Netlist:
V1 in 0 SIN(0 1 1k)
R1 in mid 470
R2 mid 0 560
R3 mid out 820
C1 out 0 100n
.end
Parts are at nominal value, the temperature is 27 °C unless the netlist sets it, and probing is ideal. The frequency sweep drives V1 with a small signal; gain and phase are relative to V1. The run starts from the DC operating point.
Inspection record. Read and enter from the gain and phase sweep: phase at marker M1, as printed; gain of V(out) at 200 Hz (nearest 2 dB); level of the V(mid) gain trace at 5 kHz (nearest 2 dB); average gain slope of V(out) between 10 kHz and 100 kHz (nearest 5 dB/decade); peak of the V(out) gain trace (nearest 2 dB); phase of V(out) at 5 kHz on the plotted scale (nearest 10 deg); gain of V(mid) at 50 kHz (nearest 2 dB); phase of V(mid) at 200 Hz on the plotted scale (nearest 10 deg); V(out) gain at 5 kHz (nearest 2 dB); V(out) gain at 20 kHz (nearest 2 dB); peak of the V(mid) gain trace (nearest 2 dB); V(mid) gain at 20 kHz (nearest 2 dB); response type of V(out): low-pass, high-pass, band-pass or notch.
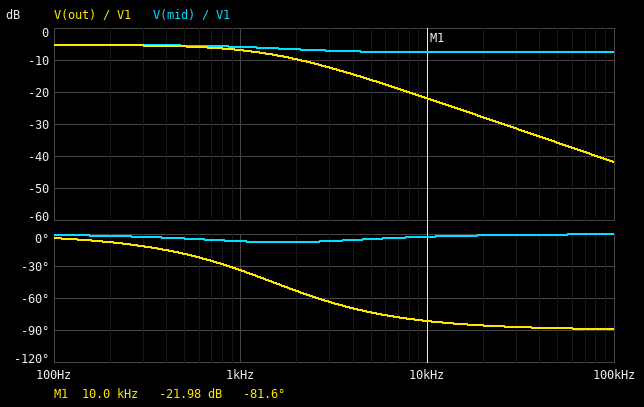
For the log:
-81.6 deg
-6 dB
-8 dB
-20 dB/decade
-6 dB
-70 deg
-8 dB
0 deg
-16 dB
-28 dB
-6 dB
-8 dB
low-pass
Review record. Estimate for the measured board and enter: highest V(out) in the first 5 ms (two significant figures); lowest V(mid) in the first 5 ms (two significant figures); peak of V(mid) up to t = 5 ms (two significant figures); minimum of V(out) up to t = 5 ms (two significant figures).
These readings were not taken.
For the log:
460 mV
-510 mV
510 mV
-450 mV
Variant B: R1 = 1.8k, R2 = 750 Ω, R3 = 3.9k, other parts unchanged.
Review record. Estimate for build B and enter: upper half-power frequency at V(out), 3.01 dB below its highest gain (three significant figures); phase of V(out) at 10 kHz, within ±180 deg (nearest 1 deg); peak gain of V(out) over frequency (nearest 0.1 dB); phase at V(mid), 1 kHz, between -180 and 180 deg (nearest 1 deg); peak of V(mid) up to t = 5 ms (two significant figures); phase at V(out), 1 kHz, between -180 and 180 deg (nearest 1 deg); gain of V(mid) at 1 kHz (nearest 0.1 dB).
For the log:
359 Hz
-88 deg
-10.6 dB
-2 deg
270 mV
-70 deg
-11.6 dB
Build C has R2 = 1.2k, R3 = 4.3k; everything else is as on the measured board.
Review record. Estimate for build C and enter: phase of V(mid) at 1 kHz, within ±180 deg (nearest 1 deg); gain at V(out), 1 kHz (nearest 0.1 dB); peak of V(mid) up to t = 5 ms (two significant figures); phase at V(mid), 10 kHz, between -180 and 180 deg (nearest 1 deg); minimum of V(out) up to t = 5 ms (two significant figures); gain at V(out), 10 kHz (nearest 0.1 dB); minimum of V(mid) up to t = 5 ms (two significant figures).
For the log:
-1 deg
-12.6 dB
680 mV
0 deg
-230 mV
-32.2 dB
-670 mV
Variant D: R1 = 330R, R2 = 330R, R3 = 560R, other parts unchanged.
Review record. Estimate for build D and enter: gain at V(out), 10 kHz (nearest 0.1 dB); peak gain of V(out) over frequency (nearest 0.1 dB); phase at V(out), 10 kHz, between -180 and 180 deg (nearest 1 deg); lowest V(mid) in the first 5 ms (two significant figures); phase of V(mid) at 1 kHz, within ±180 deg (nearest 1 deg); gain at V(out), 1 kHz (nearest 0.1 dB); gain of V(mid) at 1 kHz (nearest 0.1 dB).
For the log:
-19.4 dB
-6.0 dB
-78 deg
-480 mV
-5 deg
-6.8 dB
-6.3 dB
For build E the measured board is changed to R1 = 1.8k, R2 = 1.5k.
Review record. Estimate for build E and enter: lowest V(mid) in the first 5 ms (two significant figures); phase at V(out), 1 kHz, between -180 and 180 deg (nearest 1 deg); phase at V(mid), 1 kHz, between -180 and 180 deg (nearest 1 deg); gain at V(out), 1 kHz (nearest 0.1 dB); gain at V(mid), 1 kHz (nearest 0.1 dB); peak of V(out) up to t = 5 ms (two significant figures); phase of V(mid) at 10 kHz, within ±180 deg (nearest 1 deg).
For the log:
-360 mV
-46 deg
-19 deg
-10.0 dB
-9.0 dB
340 mV
-5 deg
